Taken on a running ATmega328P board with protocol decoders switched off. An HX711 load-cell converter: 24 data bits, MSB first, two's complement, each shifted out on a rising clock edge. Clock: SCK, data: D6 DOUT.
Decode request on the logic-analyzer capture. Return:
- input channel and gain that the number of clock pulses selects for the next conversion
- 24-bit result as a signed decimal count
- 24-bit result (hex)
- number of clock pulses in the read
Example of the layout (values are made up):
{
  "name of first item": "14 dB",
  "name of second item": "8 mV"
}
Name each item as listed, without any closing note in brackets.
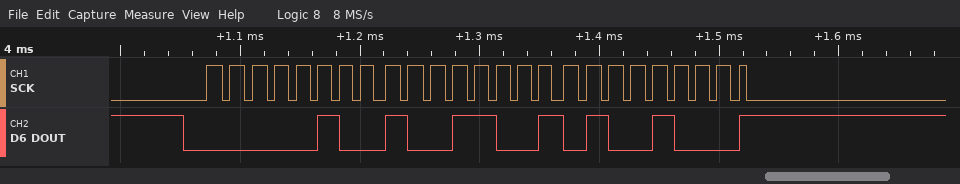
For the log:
{
  "input channel and gain that the number of clock pulses selects for the next conversion": "channel A, gain 128",
  "24-bit result as a signed decimal count": "301384",
  "24-bit result": "0x049948",
  "number of clock pulses in the read": "25"
}
